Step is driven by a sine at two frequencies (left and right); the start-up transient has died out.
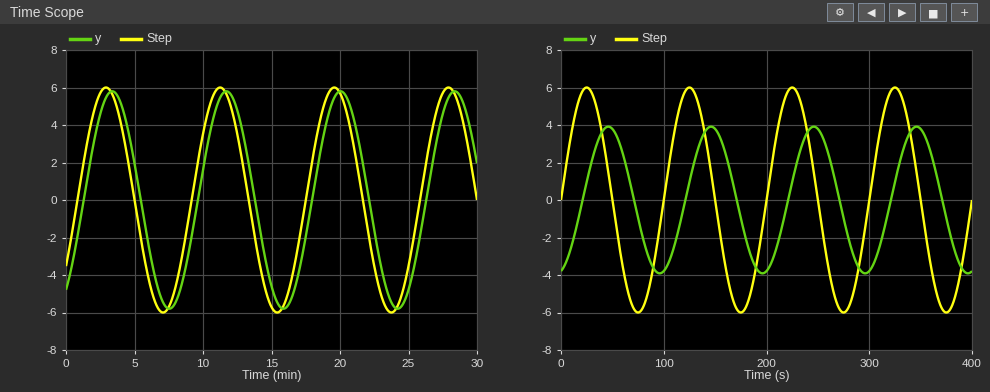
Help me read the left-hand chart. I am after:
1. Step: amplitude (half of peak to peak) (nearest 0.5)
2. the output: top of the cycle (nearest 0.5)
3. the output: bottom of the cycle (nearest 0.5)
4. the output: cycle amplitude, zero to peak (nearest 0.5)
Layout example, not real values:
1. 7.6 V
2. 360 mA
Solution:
1. 6.0
2. 6.0
3. -6.0
4. 6.0
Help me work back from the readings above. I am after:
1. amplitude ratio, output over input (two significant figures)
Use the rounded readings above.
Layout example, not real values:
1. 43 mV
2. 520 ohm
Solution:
1. 1.0
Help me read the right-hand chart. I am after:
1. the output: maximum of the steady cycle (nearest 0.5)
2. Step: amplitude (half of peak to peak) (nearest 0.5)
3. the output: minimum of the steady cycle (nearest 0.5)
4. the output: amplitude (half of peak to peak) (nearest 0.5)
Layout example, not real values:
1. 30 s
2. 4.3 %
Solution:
1. 4.0
2. 6.0
3. -4.0
4. 4.0
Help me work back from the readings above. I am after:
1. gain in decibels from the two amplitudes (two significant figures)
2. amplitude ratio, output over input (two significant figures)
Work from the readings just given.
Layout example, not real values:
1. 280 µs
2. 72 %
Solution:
1. -3.5 dB
2. 0.67
